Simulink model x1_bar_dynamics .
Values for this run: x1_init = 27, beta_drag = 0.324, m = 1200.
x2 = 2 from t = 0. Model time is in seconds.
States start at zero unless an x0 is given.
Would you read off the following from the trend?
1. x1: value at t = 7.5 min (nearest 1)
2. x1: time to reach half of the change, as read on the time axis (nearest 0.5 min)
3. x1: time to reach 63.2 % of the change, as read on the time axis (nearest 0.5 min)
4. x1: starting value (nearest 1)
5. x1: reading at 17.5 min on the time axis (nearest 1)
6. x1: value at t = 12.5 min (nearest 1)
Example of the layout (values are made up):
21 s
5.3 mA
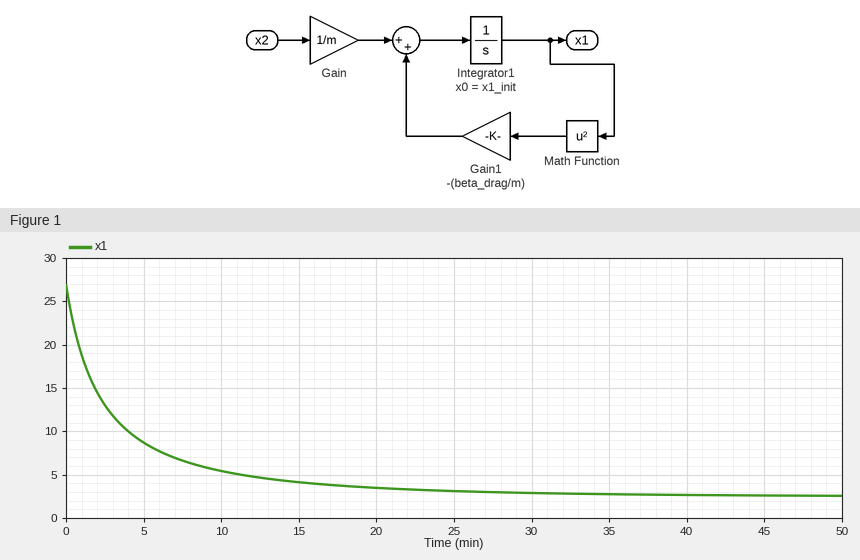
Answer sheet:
7
2.0 min
3.0 min
27
4
5
